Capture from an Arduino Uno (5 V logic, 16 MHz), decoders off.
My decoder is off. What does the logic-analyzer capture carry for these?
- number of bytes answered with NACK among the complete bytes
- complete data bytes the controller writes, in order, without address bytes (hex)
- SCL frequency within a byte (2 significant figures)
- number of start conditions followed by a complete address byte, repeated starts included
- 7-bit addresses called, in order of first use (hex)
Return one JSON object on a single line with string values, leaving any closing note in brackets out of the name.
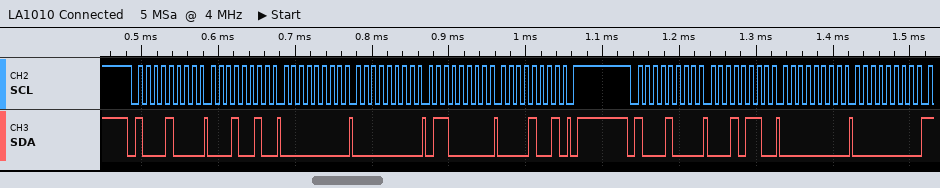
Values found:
{"number of bytes answered with NACK among the complete bytes": "0", "complete data bytes the controller writes, in order, without address bytes": "12 00 00 60 09 16 00 00", "SCL frequency within a byte": "100 kHz", "number of start conditions followed by a complete address byte, repeated starts included": "2", "7-bit addresses called, in order of first use": "0x44"}
